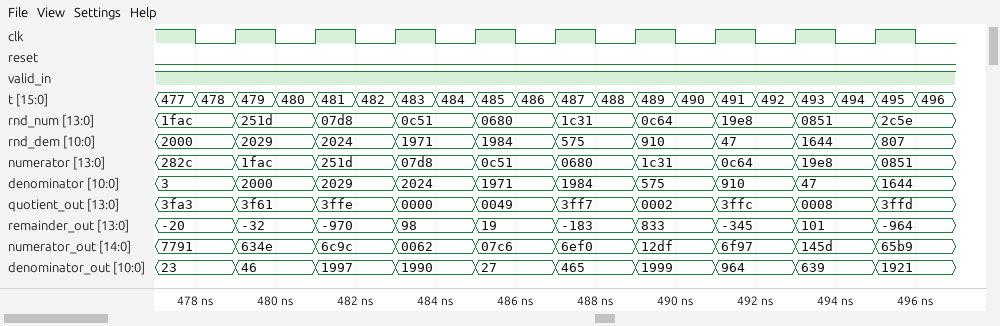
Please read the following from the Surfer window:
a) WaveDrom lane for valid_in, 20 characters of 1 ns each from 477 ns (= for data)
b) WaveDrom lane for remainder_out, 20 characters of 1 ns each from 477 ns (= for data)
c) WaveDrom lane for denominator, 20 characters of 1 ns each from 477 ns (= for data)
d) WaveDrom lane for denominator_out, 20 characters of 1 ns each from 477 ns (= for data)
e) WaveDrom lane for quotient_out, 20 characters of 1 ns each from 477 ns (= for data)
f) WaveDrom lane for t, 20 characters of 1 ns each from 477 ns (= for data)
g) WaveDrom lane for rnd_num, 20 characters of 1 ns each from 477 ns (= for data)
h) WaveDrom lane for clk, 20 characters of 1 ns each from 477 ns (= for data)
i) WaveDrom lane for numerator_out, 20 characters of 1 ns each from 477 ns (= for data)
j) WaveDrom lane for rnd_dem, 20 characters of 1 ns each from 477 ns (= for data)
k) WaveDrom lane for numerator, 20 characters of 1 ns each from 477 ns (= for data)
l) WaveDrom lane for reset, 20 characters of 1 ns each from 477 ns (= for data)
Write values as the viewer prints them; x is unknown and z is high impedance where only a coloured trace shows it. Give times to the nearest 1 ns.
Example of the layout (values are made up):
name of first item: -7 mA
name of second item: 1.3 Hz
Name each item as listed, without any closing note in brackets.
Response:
WaveDrom lane for valid_in, 20 characters of 1 ns each from 477 ns: {name: 'valid_in', wave: '1...................'}
WaveDrom lane for remainder_out, 20 characters of 1 ns each from 477 ns: {name: 'remainder_out', wave: '=.=.=.=.=.=.=.=.=.=.', data: '-20 -32 -970 98 19 -183 833 -345 101 -964'}
WaveDrom lane for denominator, 20 characters of 1 ns each from 477 ns: {name: 'denominator', wave: '=.=.=.=.=.=.=.=.=.=.', data: '3 2000 2029 2024 1971 1984 575 910 47 1644'}
WaveDrom lane for denominator_out, 20 characters of 1 ns each from 477 ns: {name: 'denominator_out', wave: '=.=.=.=.=.=.=.=.=.=.', data: '23 46 1997 1990 27 465 1999 964 639 1921'}
WaveDrom lane for quotient_out, 20 characters of 1 ns each from 477 ns: {name: 'quotient_out', wave: '=.=.=.=.=.=.=.=.=.=.', data: '3fa3 3f61 3ffe 0000 0049 3ff7 0002 3ffc 0008 3ffd'}
WaveDrom lane for t, 20 characters of 1 ns each from 477 ns: {name: 't', wave: '====================', data: '477 478 479 480 481 482 483 484 485 486 487 488 489 490 491 492 493 494 495 496'}
WaveDrom lane for rnd_num, 20 characters of 1 ns each from 477 ns: {name: 'rnd_num', wave: '=.=.=.=.=.=.=.=.=.=.', data: '1fac 251d 07d8 0c51 0680 1c31 0c64 19e8 0851 2c5e'}
WaveDrom lane for clk, 20 characters of 1 ns each from 477 ns: {name: 'clk', wave: '10101010101010101010'}
WaveDrom lane for numerator_out, 20 characters of 1 ns each from 477 ns: {name: 'numerator_out', wave: '=.=.=.=.=.=.=.=.=.=.', data: '7791 634e 6c9c 0062 07c6 6ef0 12df 6f97 145d 65b9'}
WaveDrom lane for rnd_dem, 20 characters of 1 ns each from 477 ns: {name: 'rnd_dem', wave: '=.=.=.=.=.=.=.=.=.=.', data: '2000 2029 2024 1971 1984 575 910 47 1644 807'}
WaveDrom lane for numerator, 20 characters of 1 ns each from 477 ns: {name: 'numerator', wave: '=.=.=.=.=.=.=.=.=.=.', data: '282c 1fac 251d 07d8 0c51 0680 1c31 0c64 19e8 0851'}
WaveDrom lane for reset, 20 characters of 1 ns each from 477 ns: {name: 'reset', wave: '0...................'}
